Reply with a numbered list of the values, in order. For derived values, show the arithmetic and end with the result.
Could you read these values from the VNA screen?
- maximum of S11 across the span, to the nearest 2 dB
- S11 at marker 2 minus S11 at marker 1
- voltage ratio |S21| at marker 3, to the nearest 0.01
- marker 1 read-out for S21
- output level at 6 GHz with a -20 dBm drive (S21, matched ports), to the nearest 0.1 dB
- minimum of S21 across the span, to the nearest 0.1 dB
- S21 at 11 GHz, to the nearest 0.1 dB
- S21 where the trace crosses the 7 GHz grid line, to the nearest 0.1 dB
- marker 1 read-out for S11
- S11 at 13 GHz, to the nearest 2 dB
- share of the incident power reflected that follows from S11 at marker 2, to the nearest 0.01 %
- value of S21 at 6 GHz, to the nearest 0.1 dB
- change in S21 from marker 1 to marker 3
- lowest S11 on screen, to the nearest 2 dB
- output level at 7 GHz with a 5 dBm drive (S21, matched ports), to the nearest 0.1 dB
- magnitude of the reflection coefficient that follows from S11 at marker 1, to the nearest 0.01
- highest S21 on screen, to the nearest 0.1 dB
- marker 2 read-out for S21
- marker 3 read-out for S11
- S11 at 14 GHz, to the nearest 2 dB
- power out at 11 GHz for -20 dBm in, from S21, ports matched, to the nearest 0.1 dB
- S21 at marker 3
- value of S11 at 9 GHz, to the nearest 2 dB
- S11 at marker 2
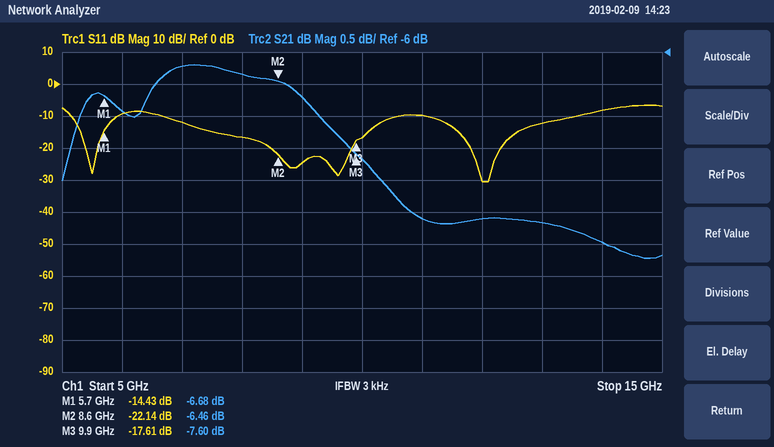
1. -6 dB
2. -22.14 − (-14.43) = -7.71 dB
3. 10^(-7.6/20) ≈ 0.42
4. -6.68 dB
5. -20 dBm + (-6.9 dB) = -26.9 dBm
6. -9.2 dB
7. -8.6 dB
8. -6.2 dB
9. -14.43 dB
10. -12 dB
11. 10^(-22.14/10) ≈ 0.61 %
12. -6.9 dB
13. -7.6 − (-6.68) = -0.92 dB
14. -30 dB
15. 5 dBm + (-6.2 dB) = -1.2 dBm
16. 10^(-14.43/20) ≈ 0.19
17. -6.2 dB
18. -6.46 dB
19. -17.61 dB
20. -8 dB
21. -20 dBm + (-8.6 dB) = -28.6 dBm
22. -7.60 dB
23. -24 dB
24. -22.14 dB
